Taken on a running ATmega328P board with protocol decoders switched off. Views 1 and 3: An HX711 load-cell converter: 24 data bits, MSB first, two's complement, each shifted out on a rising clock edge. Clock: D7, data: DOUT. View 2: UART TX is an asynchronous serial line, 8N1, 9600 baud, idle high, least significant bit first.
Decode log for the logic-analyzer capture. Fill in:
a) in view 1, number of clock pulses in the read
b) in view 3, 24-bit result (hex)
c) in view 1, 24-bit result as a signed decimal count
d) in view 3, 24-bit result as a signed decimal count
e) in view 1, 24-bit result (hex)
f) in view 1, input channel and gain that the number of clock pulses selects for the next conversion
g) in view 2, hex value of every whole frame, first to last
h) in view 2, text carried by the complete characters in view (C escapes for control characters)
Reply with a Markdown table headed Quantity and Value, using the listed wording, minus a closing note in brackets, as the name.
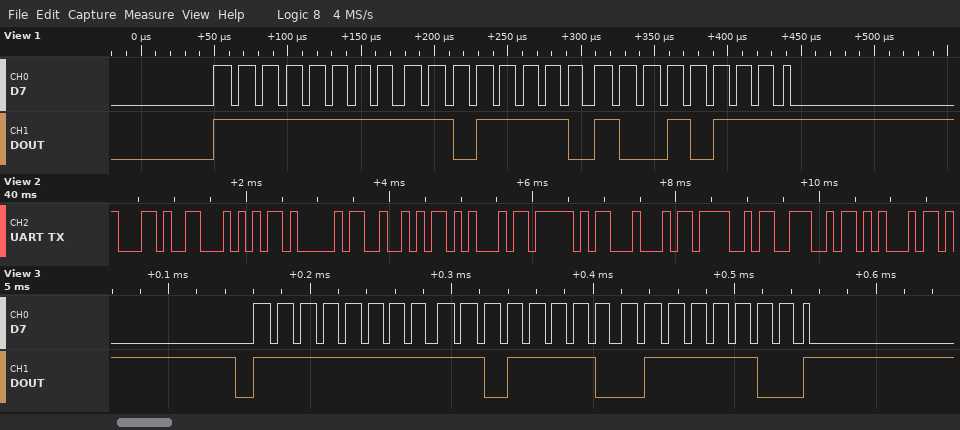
| Quantity | Value |
|---|---|
| in view 1, number of clock pulses in the read | 25 |
| in view 3, 24-bit result | 0xFFDE7C |
| in view 1, 24-bit result as a signed decimal count | -8553 |
| in view 3, 24-bit result as a signed decimal count | -8580 |
| in view 1, 24-bit result | 0xFFDE97 |
| in view 1, input channel and gain that the number of clock pulses selects for the next conversion | channel A, gain 128 |
| in view 2, hex value of every whole frame, first to last | 2C 54 41 52 45 5F 44 4F 4E 45 |
| in view 2, text carried by the complete characters in view | ",TARE_DONE" |
